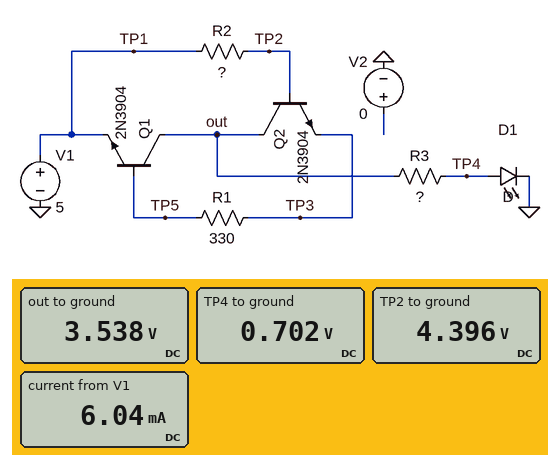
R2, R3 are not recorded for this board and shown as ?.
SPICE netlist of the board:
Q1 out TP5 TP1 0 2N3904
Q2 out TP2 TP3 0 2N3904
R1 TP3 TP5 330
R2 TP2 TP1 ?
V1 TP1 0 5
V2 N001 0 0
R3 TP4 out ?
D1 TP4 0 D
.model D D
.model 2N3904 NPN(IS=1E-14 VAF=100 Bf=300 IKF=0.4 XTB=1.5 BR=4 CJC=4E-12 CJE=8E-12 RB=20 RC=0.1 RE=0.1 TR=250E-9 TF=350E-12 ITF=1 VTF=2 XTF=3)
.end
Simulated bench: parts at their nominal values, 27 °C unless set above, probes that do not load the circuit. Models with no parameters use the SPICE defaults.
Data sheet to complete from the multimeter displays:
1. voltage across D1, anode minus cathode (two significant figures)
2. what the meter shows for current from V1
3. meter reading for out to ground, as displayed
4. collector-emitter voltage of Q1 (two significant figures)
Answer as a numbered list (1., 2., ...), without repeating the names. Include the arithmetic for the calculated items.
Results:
1. 702 mV = 700 mV
2. 6.04 mA
3. 3.538 V
4. 3.538 V - 5 V = -1.5 V
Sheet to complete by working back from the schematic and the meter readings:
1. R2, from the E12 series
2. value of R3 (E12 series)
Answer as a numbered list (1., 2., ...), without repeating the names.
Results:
1. 100 Ω
2. 470 Ω
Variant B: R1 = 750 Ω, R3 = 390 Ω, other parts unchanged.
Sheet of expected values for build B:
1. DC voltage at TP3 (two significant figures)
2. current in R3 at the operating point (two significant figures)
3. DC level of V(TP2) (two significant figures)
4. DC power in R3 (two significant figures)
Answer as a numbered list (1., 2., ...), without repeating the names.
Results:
1. 3.4 V
2. 7.0 mA
3. 4.3 V
4. 19 mW
